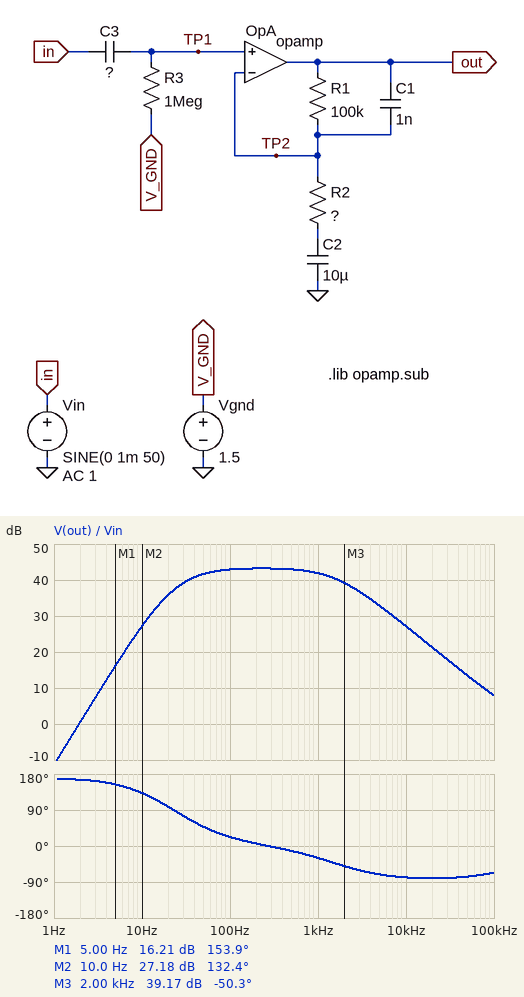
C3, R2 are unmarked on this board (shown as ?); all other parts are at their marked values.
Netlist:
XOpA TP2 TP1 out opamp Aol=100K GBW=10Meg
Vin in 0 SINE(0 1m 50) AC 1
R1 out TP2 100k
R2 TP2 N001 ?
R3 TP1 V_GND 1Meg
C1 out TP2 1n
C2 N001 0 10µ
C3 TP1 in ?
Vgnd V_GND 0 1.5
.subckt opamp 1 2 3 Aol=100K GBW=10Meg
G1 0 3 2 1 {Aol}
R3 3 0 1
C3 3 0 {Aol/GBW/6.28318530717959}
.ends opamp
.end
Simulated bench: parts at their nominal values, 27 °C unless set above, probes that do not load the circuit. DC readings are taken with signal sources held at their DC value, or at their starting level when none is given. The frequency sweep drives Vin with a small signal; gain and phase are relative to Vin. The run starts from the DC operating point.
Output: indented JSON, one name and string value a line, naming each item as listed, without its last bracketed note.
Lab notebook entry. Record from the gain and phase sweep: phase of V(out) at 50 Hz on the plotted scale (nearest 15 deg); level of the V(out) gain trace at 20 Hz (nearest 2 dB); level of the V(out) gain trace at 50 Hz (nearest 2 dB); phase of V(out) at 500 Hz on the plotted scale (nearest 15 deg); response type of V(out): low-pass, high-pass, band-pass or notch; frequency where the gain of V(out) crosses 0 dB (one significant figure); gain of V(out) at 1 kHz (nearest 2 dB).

{
  "phase of V(out) at 50 Hz on the plotted scale": "45 deg",
  "level of the V(out) gain trace at 20 Hz": "36 dB",
  "level of the V(out) gain trace at 50 Hz": "42 dB",
  "phase of V(out) at 500 Hz on the plotted scale": "-15 deg",
  "response type of V(out): low-pass, high-pass, band-pass or notch": "band-pass",
  "frequency where the gain of V(out) crosses 0 dB": "2 Hz",
  "gain of V(out) at 1 kHz": "42 dB"
}
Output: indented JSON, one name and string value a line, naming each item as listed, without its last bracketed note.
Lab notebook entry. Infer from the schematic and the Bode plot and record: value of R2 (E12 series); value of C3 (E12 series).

{
  "value of R2": "680 Ω",
  "value of C3": "6.8 nF"
}
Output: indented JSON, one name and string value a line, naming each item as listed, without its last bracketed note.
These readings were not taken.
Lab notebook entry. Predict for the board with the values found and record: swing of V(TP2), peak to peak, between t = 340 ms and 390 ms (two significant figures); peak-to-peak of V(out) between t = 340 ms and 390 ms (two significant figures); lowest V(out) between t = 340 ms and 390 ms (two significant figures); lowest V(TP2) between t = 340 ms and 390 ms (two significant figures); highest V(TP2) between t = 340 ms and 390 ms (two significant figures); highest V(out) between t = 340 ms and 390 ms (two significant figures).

{
  "swing of V(TP2), peak to peak, between t = 340 ms and 390 ms": "1.8 mV",
  "peak-to-peak of V(out) between t = 340 ms and 390 ms": "240 mV",
  "lowest V(out) between t = 340 ms and 390 ms": "1.4 V",
  "lowest V(TP2) between t = 340 ms and 390 ms": "1.5 V",
  "highest V(TP2) between t = 340 ms and 390 ms": "1.5 V",
  "highest V(out) between t = 340 ms and 390 ms": "1.6 V"
}
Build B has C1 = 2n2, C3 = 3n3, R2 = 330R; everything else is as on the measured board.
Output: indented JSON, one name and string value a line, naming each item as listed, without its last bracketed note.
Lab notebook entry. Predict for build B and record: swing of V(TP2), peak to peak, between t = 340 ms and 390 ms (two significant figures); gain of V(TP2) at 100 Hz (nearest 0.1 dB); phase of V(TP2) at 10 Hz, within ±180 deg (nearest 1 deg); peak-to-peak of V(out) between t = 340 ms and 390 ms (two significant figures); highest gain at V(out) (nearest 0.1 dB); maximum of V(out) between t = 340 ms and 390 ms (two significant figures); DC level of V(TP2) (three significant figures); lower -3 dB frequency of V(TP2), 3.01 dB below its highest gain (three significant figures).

{
  "swing of V(TP2), peak to peak, between t = 340 ms and 390 ms": "1.4 mV",
  "gain of V(TP2) at 100 Hz": "-0.9 dB",
  "phase of V(TP2) at 10 Hz, within ±180 deg": "78 deg",
  "peak-to-peak of V(out) between t = 340 ms and 390 ms": "310 mV",
  "highest gain at V(out)": "48.8 dB",
  "maximum of V(out) between t = 340 ms and 390 ms": "1.7 V",
  "DC level of V(TP2)": "1.50 V",
  "lower -3 dB frequency of V(TP2), 3.01 dB below its highest gain": "47.1 Hz"
}
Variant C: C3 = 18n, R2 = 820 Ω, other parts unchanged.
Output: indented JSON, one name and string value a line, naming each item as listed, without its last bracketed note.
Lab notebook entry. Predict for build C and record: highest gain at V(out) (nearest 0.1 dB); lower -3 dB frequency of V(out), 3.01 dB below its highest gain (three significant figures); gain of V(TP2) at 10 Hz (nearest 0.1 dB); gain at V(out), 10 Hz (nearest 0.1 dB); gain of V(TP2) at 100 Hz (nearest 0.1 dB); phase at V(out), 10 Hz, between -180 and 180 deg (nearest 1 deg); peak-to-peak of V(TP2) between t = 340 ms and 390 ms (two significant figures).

{
  "highest gain at V(out)": "41.7 dB",
  "lower -3 dB frequency of V(out), 3.01 dB below its highest gain": "22.1 Hz",
  "gain of V(TP2) at 10 Hz": "-2.5 dB",
  "gain at V(out), 10 Hz": "32.5 dB",
  "gain of V(TP2) at 100 Hz": "0 dB",
  "phase at V(out), 10 Hz, between -180 and 180 deg": "103 deg",
  "peak-to-peak of V(TP2) between t = 340 ms and 390 ms": "2.0 mV"
}
